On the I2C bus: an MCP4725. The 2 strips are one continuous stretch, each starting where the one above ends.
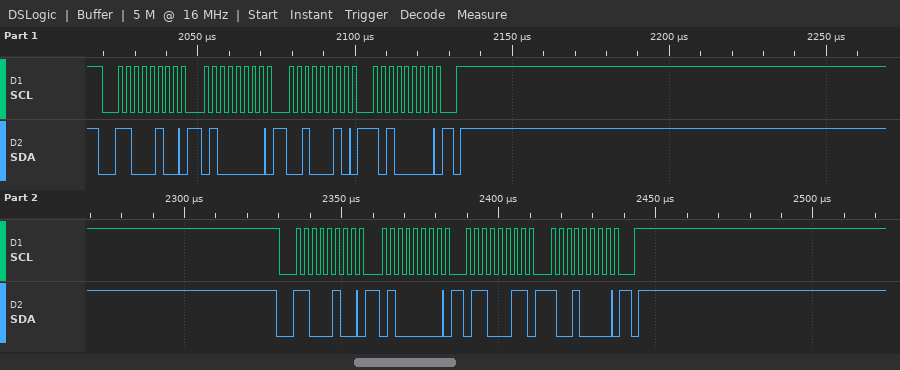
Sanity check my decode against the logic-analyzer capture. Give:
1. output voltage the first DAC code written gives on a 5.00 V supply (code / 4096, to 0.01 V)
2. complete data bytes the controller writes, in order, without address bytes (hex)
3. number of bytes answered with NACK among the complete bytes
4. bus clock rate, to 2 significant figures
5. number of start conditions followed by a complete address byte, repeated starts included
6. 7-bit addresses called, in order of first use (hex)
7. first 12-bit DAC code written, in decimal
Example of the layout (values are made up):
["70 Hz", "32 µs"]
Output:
["0.68 V", "40 22 A0 40 63 90", "0", "400 kHz", "2", "0x62", "554"]
